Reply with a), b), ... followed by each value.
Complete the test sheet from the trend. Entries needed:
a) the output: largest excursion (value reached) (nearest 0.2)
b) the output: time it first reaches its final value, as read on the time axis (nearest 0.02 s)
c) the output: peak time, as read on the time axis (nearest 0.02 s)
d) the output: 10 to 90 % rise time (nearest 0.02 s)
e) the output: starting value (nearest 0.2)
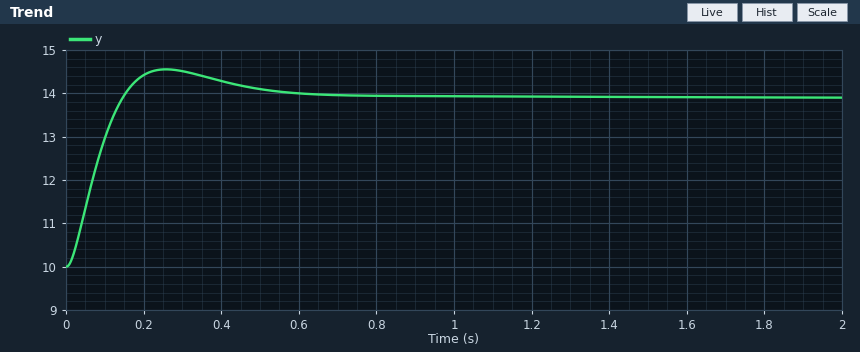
a) 14.6
b) 0.14 s
c) 0.26 s
d) 0.10 s
e) 10.0
